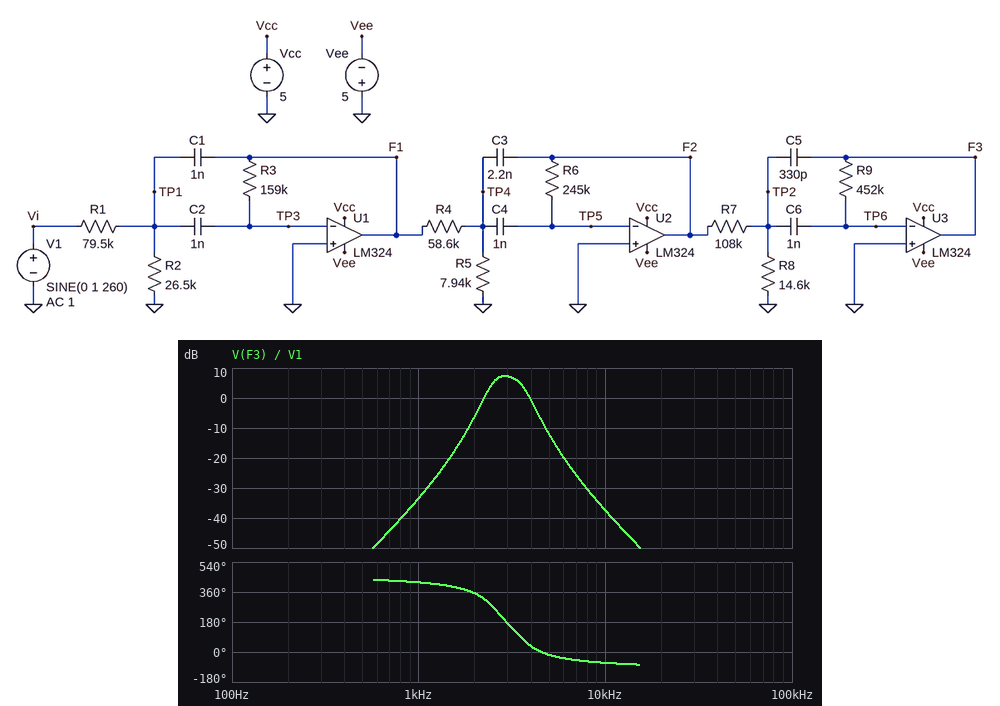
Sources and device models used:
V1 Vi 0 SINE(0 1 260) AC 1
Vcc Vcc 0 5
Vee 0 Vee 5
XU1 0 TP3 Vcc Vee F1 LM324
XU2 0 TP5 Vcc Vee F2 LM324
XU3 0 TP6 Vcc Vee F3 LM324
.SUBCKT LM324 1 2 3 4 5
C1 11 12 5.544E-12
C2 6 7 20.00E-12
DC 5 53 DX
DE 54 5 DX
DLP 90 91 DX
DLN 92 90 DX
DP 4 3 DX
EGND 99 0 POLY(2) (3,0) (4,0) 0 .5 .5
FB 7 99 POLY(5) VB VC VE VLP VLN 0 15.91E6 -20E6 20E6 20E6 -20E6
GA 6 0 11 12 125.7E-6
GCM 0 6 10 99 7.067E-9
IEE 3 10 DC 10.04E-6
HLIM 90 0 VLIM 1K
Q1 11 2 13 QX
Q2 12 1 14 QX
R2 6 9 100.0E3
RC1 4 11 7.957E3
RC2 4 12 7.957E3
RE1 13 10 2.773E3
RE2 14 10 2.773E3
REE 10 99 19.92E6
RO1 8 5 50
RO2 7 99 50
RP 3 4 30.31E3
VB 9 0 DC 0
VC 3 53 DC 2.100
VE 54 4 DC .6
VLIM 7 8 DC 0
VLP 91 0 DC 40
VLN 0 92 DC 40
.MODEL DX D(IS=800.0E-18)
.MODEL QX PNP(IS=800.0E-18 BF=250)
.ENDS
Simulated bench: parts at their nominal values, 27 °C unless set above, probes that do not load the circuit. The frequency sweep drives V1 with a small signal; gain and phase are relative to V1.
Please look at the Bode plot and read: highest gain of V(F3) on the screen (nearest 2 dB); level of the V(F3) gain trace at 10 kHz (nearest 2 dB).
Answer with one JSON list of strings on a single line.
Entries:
["8 dB", "-38 dB"]
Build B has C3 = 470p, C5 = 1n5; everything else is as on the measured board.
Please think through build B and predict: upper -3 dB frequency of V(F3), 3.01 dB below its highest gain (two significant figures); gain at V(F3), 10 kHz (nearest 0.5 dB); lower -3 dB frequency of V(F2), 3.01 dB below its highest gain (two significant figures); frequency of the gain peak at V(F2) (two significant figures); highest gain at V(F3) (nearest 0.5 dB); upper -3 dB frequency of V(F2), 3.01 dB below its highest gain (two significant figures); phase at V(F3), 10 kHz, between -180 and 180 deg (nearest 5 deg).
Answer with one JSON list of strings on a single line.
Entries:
["5.4 kHz", "-36.0 dB", "3.8 kHz", "5.2 kHz", "-9.0 dB", "6.1 kHz", "-60 deg"]
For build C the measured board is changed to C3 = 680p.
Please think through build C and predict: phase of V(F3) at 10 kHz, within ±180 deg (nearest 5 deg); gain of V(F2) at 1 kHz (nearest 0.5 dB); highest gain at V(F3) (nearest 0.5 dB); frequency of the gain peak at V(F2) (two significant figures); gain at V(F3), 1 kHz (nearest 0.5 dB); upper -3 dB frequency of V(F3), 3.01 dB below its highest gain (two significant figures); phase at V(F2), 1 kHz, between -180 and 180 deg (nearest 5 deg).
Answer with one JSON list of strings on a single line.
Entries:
["-60 deg", "-25.5 dB", "11.5 dB", "4.4 kHz", "-34.5 dB", "4.6 kHz", "160 deg"]
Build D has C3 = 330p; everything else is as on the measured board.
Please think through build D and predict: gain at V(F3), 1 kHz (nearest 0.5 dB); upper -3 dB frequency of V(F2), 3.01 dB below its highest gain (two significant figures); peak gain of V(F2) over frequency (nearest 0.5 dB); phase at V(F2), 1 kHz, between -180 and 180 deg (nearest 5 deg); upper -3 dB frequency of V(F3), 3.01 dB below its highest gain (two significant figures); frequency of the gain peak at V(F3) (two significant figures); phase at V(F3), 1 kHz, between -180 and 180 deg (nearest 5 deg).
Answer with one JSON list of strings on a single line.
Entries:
["-34.5 dB", "7.3 kHz", "1.0 dB", "160 deg", "4.5 kHz", "3.6 kHz", "65 deg"]
